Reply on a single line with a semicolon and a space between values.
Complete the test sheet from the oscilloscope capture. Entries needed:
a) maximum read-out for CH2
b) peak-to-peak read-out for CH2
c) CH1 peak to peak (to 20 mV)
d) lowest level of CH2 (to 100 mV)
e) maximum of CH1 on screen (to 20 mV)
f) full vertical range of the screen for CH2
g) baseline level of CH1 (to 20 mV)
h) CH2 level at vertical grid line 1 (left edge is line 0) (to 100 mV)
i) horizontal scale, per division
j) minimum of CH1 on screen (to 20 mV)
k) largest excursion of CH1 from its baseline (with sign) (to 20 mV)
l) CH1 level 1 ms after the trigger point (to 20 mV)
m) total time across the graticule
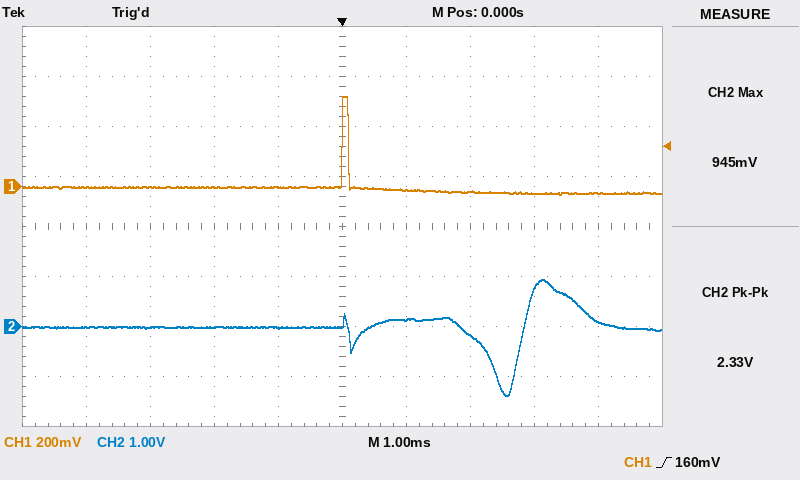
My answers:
945 mV; 2.33 V; 400 mV; -1.4 V; 360 mV; 8 V; 0 mV; 0.0 V; 1 ms; -40 mV; +360 mV; -20 mV; 10 ms
